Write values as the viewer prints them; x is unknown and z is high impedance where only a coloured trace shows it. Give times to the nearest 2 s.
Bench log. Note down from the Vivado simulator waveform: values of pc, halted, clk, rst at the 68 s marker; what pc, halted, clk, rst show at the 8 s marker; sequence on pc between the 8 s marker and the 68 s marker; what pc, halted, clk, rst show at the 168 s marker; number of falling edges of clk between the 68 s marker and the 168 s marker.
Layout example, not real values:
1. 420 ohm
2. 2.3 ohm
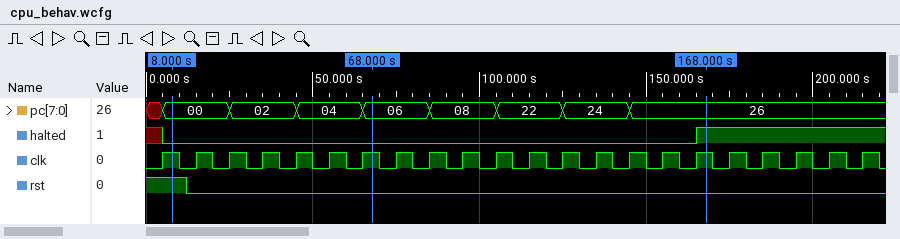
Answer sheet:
1. pc=06, halted=0, clk=1, rst=0
2. pc=00, halted=0, clk=1, rst=1
3. 00, 02, 04, 06
4. pc=26, halted=1, clk=1, rst=0
5. 10
